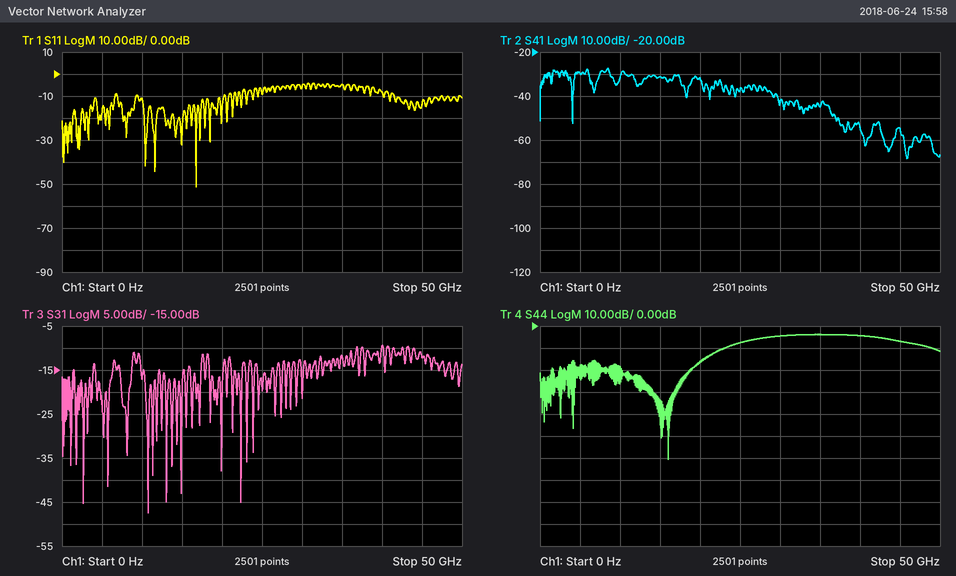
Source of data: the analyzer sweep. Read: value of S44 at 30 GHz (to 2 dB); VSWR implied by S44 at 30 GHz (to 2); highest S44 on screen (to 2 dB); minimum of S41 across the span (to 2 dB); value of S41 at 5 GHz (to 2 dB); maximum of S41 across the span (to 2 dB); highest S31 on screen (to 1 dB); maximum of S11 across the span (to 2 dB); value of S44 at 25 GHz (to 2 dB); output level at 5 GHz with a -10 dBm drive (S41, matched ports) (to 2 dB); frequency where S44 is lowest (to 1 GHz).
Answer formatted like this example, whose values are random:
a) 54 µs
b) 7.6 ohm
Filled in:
a) -4 dB
b) 4
c) -4 dB
d) -68 dB
e) -30 dB
f) -28 dB
g) -9 dB
h) -4 dB
i) -8 dB
j) -40 dBm
k) 16 GHz
